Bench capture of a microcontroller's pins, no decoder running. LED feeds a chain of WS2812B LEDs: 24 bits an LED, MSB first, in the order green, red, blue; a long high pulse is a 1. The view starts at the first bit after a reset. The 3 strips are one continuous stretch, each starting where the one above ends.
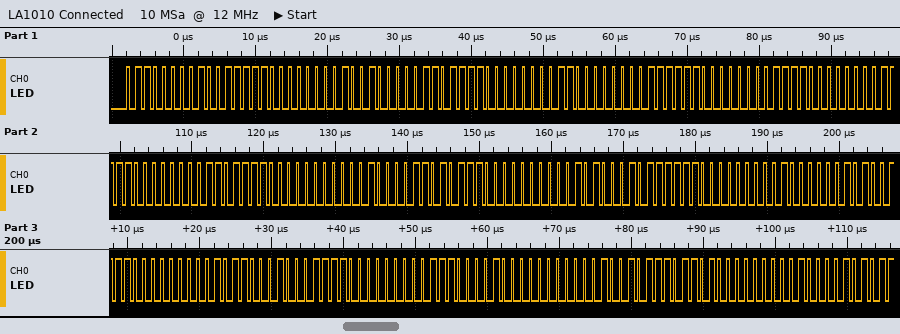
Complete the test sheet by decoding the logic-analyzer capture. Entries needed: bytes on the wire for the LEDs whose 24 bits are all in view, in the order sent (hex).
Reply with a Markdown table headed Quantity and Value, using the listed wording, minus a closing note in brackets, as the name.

| Quantity | Value |
|---|---|
| bytes on the wire for the LEDs whose 24 bits are all in view, in the order sent | 60 9F 00 90 6F 00 C0 3F 00 F0 0F 00 DE 00 21 AE 00 51 7E 00 81 4E 00 B1 1E 00 E1 00 12 ED |
